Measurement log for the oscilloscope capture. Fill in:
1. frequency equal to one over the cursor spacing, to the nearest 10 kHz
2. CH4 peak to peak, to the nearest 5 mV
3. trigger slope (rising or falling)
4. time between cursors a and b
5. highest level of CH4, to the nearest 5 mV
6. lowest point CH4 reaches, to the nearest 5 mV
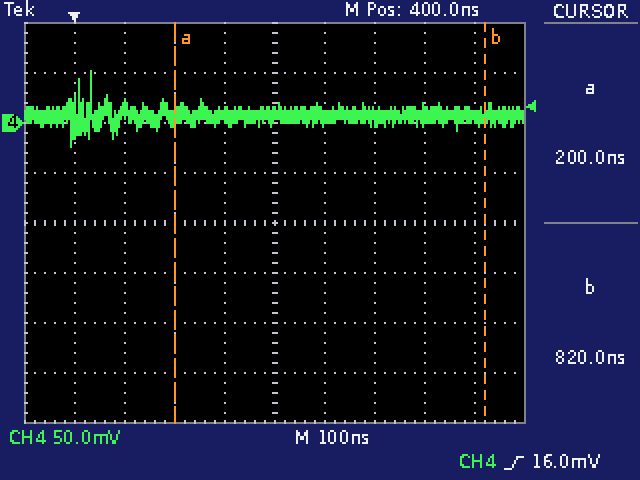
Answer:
1.61 MHz
75 mV
rising
620 ns
50 mV
-25 mV
